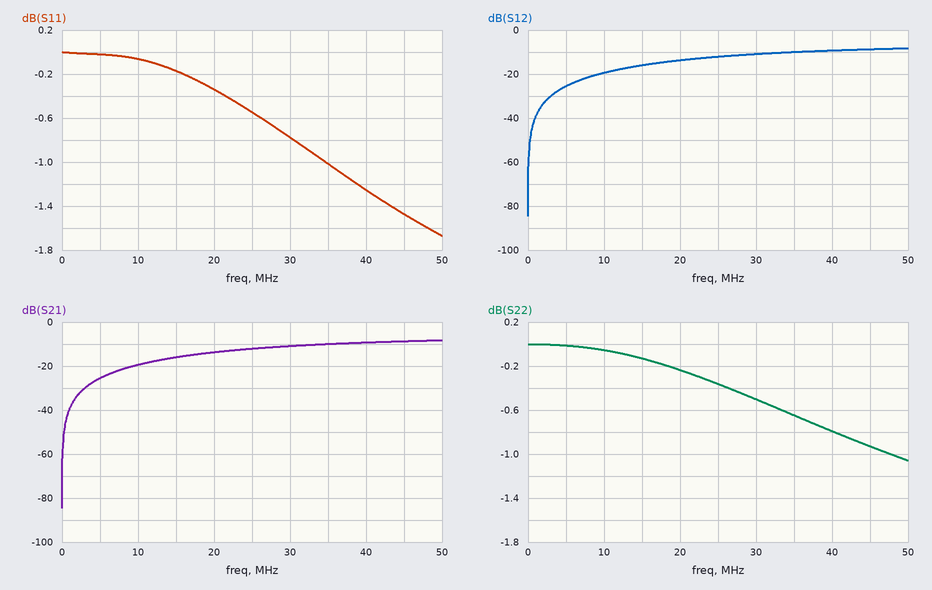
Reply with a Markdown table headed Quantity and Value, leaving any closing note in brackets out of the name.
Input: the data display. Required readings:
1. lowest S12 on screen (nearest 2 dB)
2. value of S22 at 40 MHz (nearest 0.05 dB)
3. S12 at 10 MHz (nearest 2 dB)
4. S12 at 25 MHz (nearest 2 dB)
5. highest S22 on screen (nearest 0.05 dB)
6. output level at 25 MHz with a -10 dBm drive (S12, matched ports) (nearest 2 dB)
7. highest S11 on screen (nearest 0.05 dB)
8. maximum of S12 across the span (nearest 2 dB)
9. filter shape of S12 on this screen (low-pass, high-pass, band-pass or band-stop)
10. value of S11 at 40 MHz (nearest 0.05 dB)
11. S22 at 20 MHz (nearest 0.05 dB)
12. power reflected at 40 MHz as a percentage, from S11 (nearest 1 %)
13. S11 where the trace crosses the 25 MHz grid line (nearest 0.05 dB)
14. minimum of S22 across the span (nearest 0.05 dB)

| Quantity | Value |
|---|---|
| lowest S12 on screen | -84 dB |
| value of S22 at 40 MHz | -0.80 dB |
| S12 at 10 MHz | -20 dB |
| S12 at 25 MHz | -12 dB |
| highest S22 on screen | 0.00 dB |
| output level at 25 MHz with a -10 dBm drive (S12, matched ports) | -22 dBm |
| highest S11 on screen | 0.00 dB |
| maximum of S12 across the span | -8 dB |
| filter shape of S12 on this screen | high-pass |
| value of S11 at 40 MHz | -1.25 dB |
| S22 at 20 MHz | -0.25 dB |
| power reflected at 40 MHz as a percentage, from S11 | 75 % |
| S11 where the trace crosses the 25 MHz grid line | -0.55 dB |
| minimum of S22 across the span | -1.05 dB |
